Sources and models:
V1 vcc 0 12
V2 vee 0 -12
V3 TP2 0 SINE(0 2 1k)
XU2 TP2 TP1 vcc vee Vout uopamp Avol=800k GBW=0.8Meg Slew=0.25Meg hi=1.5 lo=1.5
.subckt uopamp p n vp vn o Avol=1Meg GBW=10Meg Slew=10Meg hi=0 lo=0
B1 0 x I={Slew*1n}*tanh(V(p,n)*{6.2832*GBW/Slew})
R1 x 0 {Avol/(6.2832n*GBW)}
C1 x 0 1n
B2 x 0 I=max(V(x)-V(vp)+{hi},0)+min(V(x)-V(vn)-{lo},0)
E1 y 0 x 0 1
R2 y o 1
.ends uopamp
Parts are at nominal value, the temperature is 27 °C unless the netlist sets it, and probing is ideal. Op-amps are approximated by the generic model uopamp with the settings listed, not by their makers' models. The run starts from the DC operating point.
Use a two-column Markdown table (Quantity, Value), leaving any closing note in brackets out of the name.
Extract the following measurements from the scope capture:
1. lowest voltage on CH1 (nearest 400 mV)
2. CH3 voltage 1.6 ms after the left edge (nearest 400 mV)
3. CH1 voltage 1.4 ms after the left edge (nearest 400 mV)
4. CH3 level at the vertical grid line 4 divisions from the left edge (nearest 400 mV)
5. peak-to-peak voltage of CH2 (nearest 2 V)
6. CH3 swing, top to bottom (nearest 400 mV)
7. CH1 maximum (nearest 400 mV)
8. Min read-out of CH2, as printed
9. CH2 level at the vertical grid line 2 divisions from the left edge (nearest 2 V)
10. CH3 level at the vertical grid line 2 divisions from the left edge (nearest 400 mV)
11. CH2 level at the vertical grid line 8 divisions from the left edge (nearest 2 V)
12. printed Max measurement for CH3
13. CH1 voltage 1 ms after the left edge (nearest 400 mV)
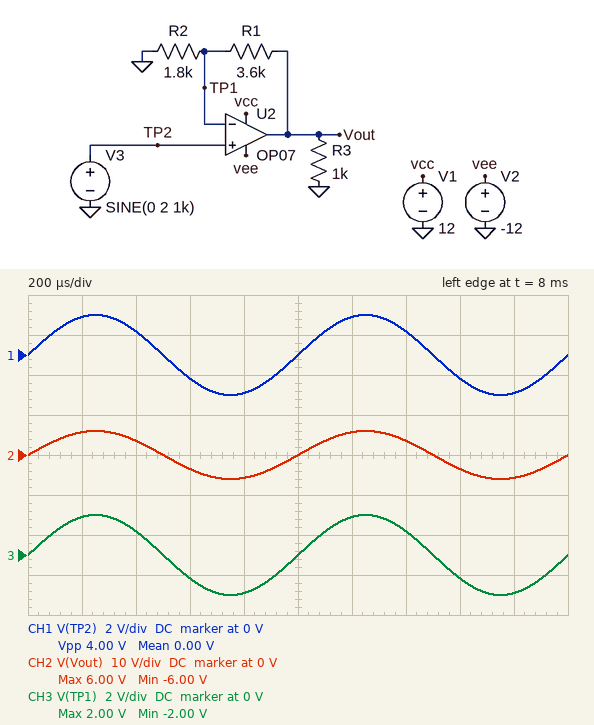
| Quantity | Value |
|---|---|
| lowest voltage on CH1 | -2.0 V |
| CH3 voltage 1.6 ms after the left edge | -1.2 V |
| CH1 voltage 1.4 ms after the left edge | 1.2 V |
| CH3 level at the vertical grid line 4 divisions from the left edge | -2.0 V |
| peak-to-peak voltage of CH2 | 12 V |
| CH3 swing, top to bottom | 4.0 V |
| CH1 maximum | 2.0 V |
| Min read-out of CH2, as printed | -6.00 V |
| CH2 level at the vertical grid line 2 divisions from the left edge | 4 V |
| CH3 level at the vertical grid line 2 divisions from the left edge | 1.2 V |
| CH2 level at the vertical grid line 8 divisions from the left edge | -4 V |
| printed Max measurement for CH3 | 2.00 V |
| CH1 voltage 1 ms after the left edge | 0 V |
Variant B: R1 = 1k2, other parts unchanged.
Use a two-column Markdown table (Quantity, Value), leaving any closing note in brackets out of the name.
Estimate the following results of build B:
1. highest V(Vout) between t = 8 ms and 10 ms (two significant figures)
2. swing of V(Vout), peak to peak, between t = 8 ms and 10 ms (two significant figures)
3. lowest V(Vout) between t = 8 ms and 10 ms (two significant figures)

| Quantity | Value |
|---|---|
| highest V(Vout) between t = 8 ms and 10 ms | 3.3 V |
| swing of V(Vout), peak to peak, between t = 8 ms and 10 ms | 6.7 V |
| lowest V(Vout) between t = 8 ms and 10 ms | -3.3 V |
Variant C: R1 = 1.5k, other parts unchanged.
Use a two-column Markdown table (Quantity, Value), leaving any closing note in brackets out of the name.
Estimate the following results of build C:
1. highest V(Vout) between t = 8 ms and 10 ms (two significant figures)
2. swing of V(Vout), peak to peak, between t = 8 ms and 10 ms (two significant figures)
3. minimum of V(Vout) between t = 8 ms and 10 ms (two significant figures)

| Quantity | Value |
|---|---|
| highest V(Vout) between t = 8 ms and 10 ms | 3.7 V |
| swing of V(Vout), peak to peak, between t = 8 ms and 10 ms | 7.3 V |
| minimum of V(Vout) between t = 8 ms and 10 ms | -3.7 V |
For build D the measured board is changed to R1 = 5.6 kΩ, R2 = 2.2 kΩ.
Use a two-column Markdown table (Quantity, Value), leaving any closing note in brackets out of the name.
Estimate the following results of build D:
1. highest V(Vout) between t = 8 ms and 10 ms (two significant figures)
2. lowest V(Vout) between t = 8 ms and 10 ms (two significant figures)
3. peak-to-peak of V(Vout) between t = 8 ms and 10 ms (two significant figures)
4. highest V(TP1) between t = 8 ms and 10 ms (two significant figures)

| Quantity | Value |
|---|---|
| highest V(Vout) between t = 8 ms and 10 ms | 7.1 V |
| lowest V(Vout) between t = 8 ms and 10 ms | -7.1 V |
| peak-to-peak of V(Vout) between t = 8 ms and 10 ms | 14 V |
| highest V(TP1) between t = 8 ms and 10 ms | 2.0 V |
